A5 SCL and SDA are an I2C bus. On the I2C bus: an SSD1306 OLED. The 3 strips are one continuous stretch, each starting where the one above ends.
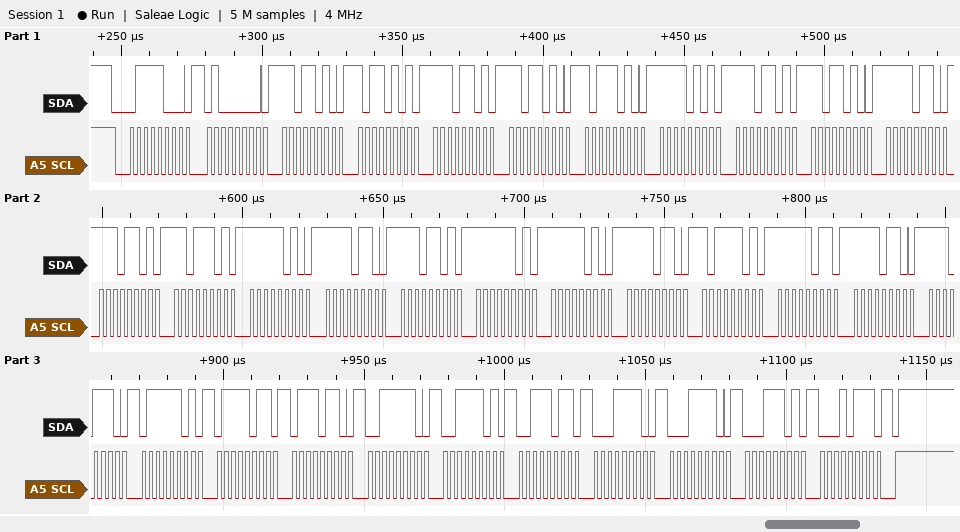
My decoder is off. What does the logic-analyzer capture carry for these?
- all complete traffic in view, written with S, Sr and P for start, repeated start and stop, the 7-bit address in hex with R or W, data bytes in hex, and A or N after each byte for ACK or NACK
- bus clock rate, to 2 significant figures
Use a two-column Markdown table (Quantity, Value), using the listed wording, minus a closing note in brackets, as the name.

| Quantity | Value |
|---|---|
| all complete traffic in view, written with S, Sr and P for start, repeated start and stop, the 7-bit address in hex with R or W, data bytes in hex, and A or N after each byte for ACK or NACK | S 3CW A 40 A DA A B5 A ED A DA A BA A F5 A ED A DA A F6 A ED A DD A FA A F6 A ED A FD A FA A F6 A BD A FB A F6 A EE A 7D A 7B A 76 A 3E A 3D A 3B A 1E A 1E A 1D A 17 A P |
| bus clock rate, to 2 significant figures | 400 kHz |
